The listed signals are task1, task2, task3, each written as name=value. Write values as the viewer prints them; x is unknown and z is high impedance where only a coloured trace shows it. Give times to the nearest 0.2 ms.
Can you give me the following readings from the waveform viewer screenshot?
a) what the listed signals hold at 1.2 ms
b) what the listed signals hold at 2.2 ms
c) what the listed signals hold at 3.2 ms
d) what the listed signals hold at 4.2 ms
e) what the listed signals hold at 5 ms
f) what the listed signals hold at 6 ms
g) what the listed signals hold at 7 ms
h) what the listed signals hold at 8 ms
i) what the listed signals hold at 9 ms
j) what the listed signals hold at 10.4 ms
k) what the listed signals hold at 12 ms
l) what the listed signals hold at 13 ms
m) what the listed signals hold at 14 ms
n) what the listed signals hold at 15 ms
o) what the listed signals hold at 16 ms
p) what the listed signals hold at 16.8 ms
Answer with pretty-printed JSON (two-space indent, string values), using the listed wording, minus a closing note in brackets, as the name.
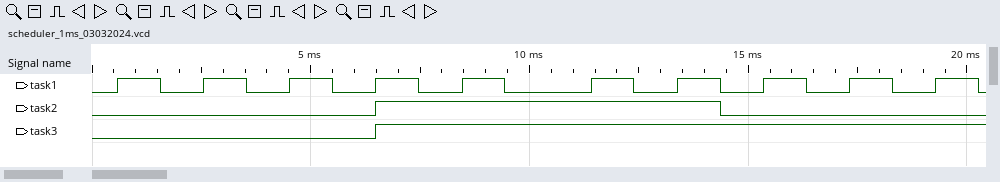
{
  "what the listed signals hold at 1.2 ms": "task1=1, task2=0, task3=0",
  "what the listed signals hold at 2.2 ms": "task1=0, task2=0, task3=0",
  "what the listed signals hold at 3.2 ms": "task1=1, task2=0, task3=0",
  "what the listed signals hold at 4.2 ms": "task1=0, task2=0, task3=0",
  "what the listed signals hold at 5 ms": "task1=1, task2=0, task3=0",
  "what the listed signals hold at 6 ms": "task1=0, task2=0, task3=0",
  "what the listed signals hold at 7 ms": "task1=1, task2=1, task3=1",
  "what the listed signals hold at 8 ms": "task1=0, task2=1, task3=1",
  "what the listed signals hold at 9 ms": "task1=1, task2=1, task3=1",
  "what the listed signals hold at 10.4 ms": "task1=0, task2=1, task3=1",
  "what the listed signals hold at 12 ms": "task1=1, task2=1, task3=1",
  "what the listed signals hold at 13 ms": "task1=0, task2=1, task3=1",
  "what the listed signals hold at 14 ms": "task1=1, task2=1, task3=1",
  "what the listed signals hold at 15 ms": "task1=0, task2=0, task3=1",
  "what the listed signals hold at 16 ms": "task1=1, task2=0, task3=1",
  "what the listed signals hold at 16.8 ms": "task1=0, task2=0, task3=1"
}
